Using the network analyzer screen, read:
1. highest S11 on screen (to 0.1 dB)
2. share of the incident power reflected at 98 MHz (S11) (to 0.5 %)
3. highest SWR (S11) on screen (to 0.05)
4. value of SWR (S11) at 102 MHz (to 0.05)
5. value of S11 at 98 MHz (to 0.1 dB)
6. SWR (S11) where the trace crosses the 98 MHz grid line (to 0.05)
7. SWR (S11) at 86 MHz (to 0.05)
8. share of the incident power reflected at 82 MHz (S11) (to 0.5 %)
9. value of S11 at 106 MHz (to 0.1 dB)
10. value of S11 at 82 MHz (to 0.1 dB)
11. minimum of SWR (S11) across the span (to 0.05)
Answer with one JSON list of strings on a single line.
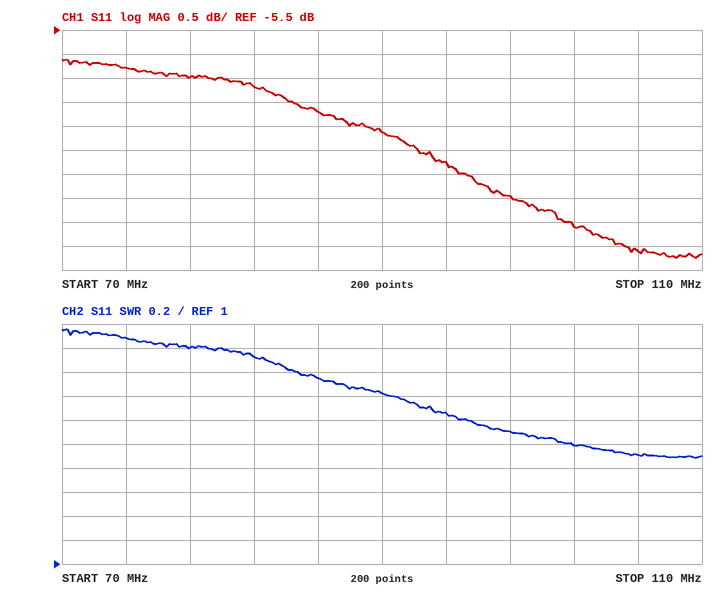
["-6.1 dB", "12.5 %", "2.95", "2.00", "-9.0 dB", "2.10", "2.55", "21.5 %", "-10.1 dB", "-6.7 dB", "1.90"]
